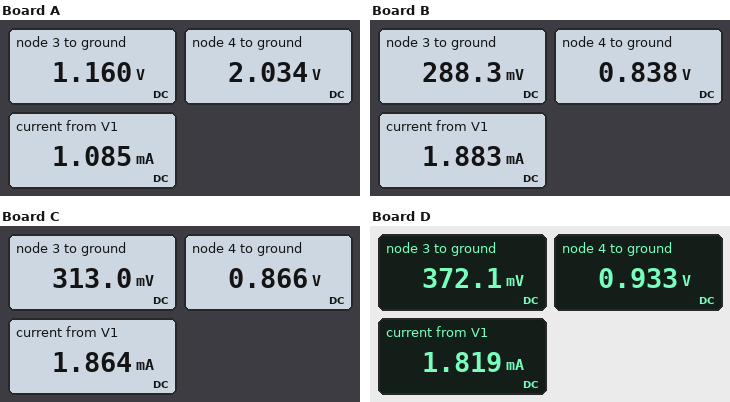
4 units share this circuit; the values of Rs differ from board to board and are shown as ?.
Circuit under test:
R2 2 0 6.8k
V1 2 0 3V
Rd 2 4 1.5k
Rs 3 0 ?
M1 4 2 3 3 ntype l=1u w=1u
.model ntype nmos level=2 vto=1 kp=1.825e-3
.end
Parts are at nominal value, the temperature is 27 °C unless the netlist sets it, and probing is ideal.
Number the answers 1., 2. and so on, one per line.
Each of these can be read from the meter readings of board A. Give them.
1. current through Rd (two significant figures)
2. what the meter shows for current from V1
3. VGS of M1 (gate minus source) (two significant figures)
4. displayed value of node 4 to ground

1. 640 µA
2. 1.085 mA
3. 1.8 V
4. 2.034 V
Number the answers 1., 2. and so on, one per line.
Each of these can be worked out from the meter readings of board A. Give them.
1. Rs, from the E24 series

1. 1.8 kΩ
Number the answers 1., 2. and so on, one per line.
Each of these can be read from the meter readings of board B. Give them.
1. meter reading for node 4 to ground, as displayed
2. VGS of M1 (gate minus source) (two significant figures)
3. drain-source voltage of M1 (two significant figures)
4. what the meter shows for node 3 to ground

1. 0.838 V
2. 2.7 V
3. 550 mV
4. 288.3 mV
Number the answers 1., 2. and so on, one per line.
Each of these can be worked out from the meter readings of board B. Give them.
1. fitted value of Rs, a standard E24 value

1. 200 Ω
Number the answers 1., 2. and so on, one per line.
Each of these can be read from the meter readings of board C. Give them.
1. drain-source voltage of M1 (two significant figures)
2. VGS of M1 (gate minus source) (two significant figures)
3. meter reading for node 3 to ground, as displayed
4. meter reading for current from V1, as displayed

1. 550 mV
2. 2.7 V
3. 313.0 mV
4. 1.864 mA
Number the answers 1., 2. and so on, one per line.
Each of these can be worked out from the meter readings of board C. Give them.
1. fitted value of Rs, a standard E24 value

1. 220 Ω
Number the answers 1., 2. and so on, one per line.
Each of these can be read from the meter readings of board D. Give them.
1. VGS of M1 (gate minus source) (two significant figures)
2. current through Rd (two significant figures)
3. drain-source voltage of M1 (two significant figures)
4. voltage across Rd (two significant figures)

1. 2.6 V
2. 1.4 mA
3. 560 mV
4. 2.1 V
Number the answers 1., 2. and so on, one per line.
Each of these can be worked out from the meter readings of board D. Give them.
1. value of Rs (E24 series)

1. 270 Ω
